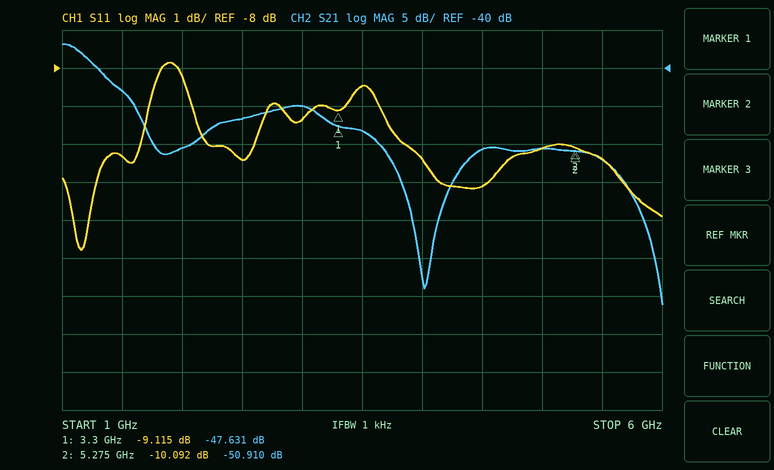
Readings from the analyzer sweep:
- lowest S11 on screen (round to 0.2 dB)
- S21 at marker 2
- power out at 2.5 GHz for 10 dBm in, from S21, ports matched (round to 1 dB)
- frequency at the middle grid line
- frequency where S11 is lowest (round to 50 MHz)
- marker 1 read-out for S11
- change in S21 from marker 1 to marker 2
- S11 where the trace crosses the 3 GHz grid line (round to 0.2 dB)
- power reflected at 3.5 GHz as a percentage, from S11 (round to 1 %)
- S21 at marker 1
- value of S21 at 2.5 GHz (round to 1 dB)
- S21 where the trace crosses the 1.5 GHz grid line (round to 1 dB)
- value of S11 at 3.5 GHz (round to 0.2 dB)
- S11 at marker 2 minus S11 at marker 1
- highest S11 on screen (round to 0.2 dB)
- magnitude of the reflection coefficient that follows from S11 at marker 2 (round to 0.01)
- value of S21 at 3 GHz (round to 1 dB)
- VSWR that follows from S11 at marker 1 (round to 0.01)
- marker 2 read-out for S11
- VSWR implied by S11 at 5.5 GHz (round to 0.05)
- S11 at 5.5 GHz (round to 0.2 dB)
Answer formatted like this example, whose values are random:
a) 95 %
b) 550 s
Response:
a) -12.8 dB
b) -50.910 dB
c) -37 dBm
d) 3.5 GHz
e) 1.15 GHz
f) -9.115 dB
g) -3.279 dB
h) -9.4 dB
i) 14 %
j) -47.631 dB
k) -47 dB
l) -43 dB
m) -8.4 dB
n) -0.977 dB
o) -7.8 dB
p) 0.31
q) -45 dB
r) 2.08
s) -10.092 dB
t) 1.85
u) -10.4 dB
